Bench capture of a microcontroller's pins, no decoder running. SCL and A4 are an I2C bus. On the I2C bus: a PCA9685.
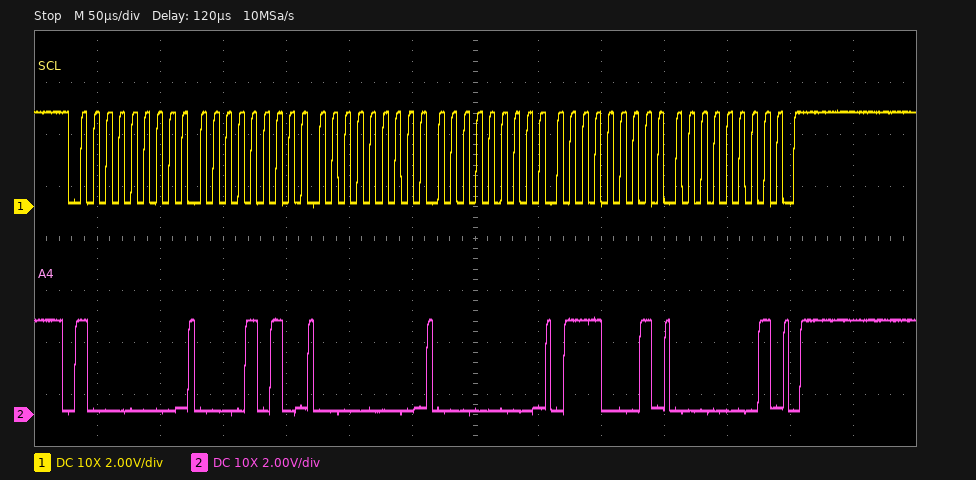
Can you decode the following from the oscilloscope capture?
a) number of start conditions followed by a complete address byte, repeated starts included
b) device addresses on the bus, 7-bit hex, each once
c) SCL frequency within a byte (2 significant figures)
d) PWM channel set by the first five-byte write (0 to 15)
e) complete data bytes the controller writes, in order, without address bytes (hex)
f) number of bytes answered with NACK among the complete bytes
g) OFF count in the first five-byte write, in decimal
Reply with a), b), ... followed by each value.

a) 1
b) 0x40
c) 100 kHz
d) 1
e) 0A 00 00 71 01
f) 0
g) 369
